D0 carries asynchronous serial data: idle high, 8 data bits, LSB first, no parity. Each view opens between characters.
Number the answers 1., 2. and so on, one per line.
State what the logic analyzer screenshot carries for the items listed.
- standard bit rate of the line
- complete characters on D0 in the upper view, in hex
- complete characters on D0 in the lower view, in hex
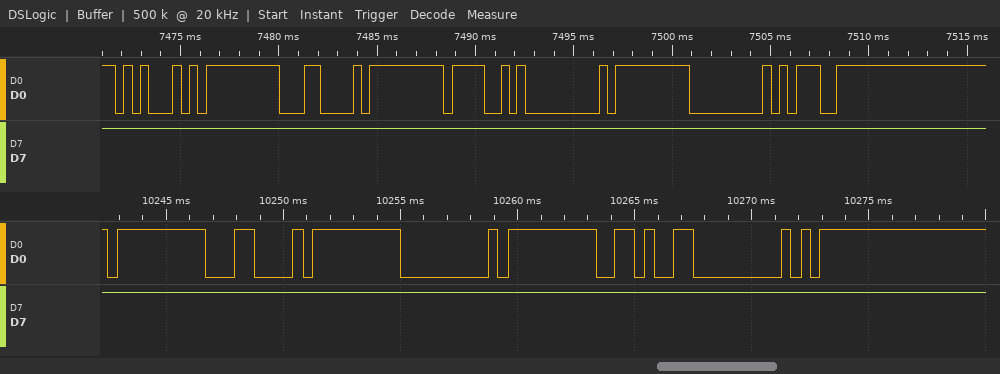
1. 2400 baud
2. 45, FF, 0C, FF, 4F, 00, FF, 00, 9D
3. FF, 0C, FF, 00, FF, 96, 00, FD
